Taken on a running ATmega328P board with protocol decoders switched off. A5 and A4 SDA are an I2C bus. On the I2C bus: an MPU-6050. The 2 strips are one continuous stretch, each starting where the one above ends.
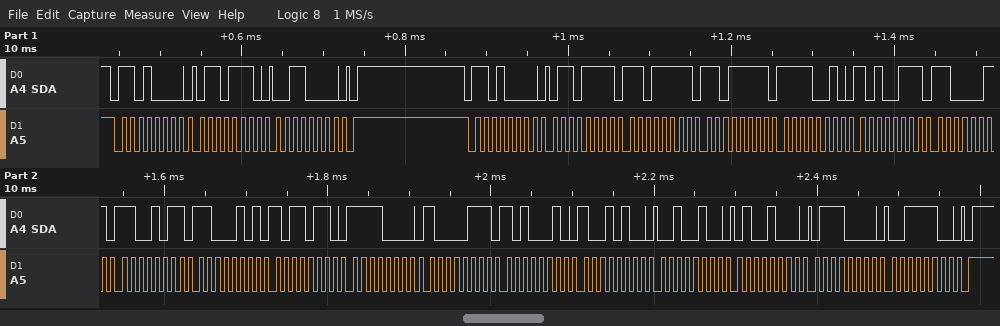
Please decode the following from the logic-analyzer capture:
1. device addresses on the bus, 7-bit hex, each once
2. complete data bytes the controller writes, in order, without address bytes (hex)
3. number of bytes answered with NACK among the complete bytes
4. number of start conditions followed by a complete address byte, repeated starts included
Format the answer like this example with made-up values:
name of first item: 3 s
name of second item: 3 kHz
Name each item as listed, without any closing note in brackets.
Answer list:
device addresses on the bus, 7-bit hex, each once: 0x68
complete data bytes the controller writes, in order, without address bytes: 6E 30 6F DF DF F2 A7 C3 CB C5 B6 F0 87 A2 94 24 48 70 3C
number of bytes answered with NACK among the complete bytes: 0
number of start conditions followed by a complete address byte, repeated starts included: 2
